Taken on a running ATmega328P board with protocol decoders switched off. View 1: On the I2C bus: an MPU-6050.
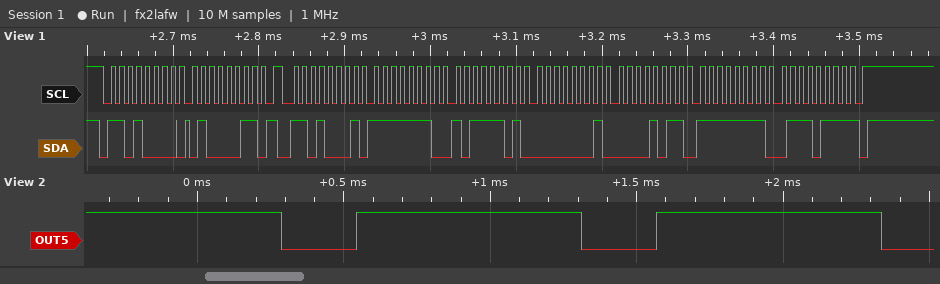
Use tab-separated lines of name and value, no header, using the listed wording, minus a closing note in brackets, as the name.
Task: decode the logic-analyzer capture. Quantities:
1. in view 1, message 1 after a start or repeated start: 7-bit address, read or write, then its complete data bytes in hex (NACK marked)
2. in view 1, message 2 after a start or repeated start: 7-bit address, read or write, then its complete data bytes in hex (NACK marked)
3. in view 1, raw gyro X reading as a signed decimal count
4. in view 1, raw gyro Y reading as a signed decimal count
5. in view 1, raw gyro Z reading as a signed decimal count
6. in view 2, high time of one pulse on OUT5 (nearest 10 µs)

in view 1, message 1 after a start or repeated start: 7-bit address, read or write, then its complete data bytes in hex	0x68 write: 43
in view 1, message 2 after a start or repeated start: 7-bit address, read or write, then its complete data bytes in hex	0x68 read: FE BD 01 0B FF 77 NACK
in view 1, raw gyro X reading as a signed decimal count	-323
in view 1, raw gyro Y reading as a signed decimal count	267
in view 1, raw gyro Z reading as a signed decimal count	-137
in view 2, high time of one pulse on OUT5	770 µs
